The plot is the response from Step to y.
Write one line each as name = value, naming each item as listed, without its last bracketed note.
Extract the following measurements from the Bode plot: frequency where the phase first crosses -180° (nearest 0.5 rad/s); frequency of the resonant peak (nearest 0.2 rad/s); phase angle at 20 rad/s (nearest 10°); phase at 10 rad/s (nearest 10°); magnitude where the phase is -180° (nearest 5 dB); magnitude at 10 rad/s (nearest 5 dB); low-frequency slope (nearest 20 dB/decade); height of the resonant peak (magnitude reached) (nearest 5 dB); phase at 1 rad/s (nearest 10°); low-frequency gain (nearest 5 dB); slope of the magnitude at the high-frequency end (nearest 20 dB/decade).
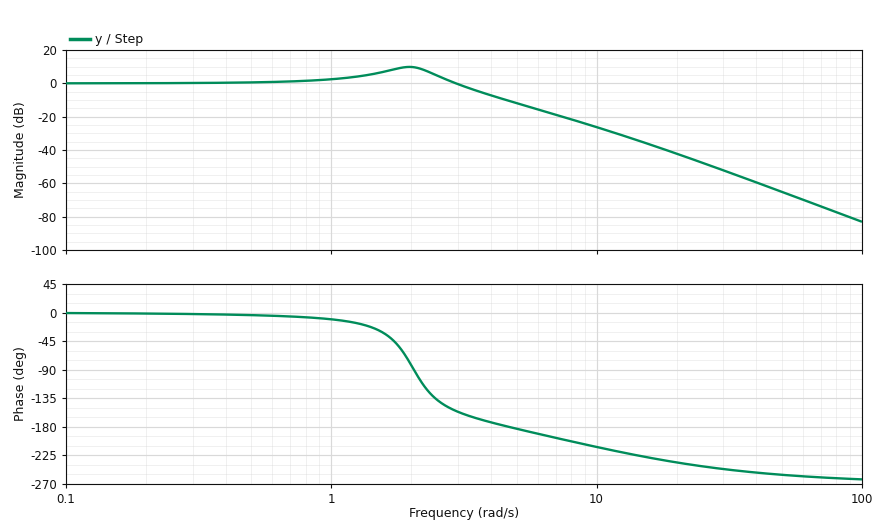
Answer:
frequency where the phase first crosses -180° = 4.5 rad/s
frequency of the resonant peak = 2.0 rad/s
phase angle at 20 rad/s = -240°
phase at 10 rad/s = -210°
magnitude where the phase is -180° = -10 dB
magnitude at 10 rad/s = -25 dB
low-frequency slope = 0 dB/decade
height of the resonant peak (magnitude reached) = 10 dB
phase at 1 rad/s = -10°
low-frequency gain = 0 dB
slope of the magnitude at the high-frequency end = -60 dB/decade
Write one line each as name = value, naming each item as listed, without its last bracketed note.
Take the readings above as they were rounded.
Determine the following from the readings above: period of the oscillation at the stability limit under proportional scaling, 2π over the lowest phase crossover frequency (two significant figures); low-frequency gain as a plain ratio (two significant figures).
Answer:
period of the oscillation at the stability limit under proportional scaling, 2π over the lowest phase crossover frequency = 1.4 s
low-frequency gain as a plain ratio = 1.0
